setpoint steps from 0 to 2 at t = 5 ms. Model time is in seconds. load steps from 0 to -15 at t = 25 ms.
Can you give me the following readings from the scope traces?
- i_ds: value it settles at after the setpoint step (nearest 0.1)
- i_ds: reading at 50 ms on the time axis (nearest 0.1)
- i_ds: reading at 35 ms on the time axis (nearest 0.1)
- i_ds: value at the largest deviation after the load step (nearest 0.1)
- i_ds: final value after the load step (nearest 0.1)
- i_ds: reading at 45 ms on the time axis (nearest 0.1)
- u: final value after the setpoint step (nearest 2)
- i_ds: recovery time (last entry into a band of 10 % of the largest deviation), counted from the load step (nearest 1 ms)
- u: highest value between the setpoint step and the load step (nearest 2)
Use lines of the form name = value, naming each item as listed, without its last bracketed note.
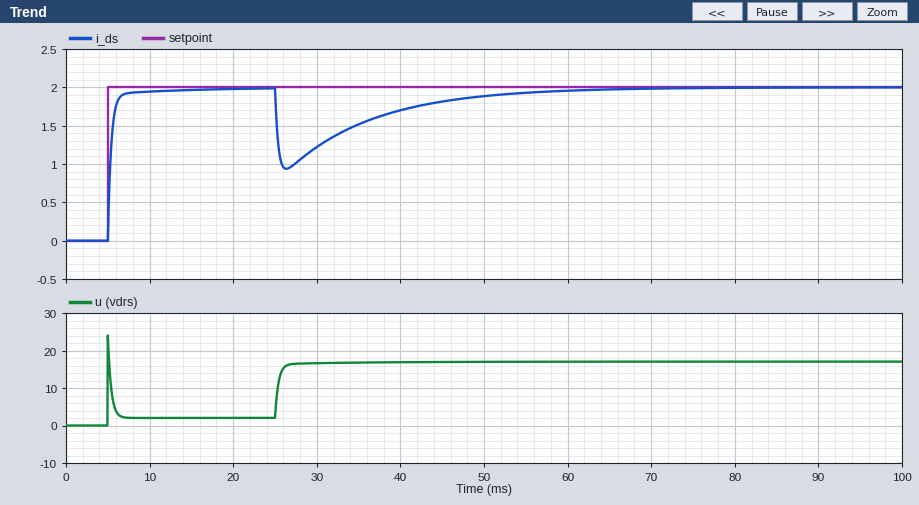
i_ds: value it settles at after the setpoint step = 2.0
i_ds: reading at 50 ms on the time axis = 1.9
i_ds: reading at 35 ms on the time axis = 1.5
i_ds: value at the largest deviation after the load step = 0.9
i_ds: final value after the load step = 2.0
i_ds: reading at 45 ms on the time axis = 1.8
u: final value after the setpoint step = 2
i_ds: recovery time (last entry into a band of 10 % of the largest deviation), counted from the load step = 26 ms
u: highest value between the setpoint step and the load step = 24
